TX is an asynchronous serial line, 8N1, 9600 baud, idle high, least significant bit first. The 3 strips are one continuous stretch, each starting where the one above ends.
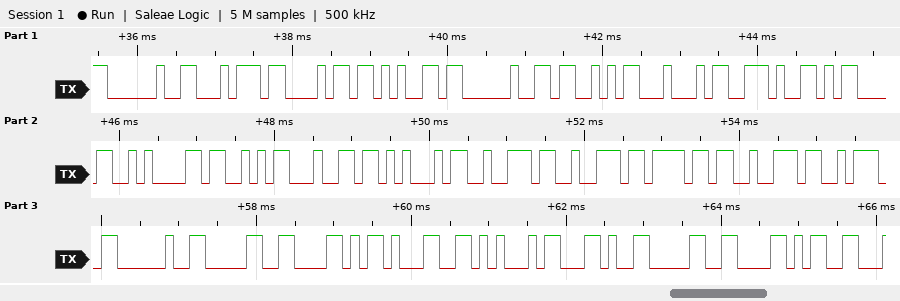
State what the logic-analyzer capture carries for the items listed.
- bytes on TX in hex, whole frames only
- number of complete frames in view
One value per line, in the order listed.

20 74 68 65 20 53 44 2E 0D 0A 53 64 45 72 72 6F 72 3A 20 30 58 31 45 2C 30 58
26
